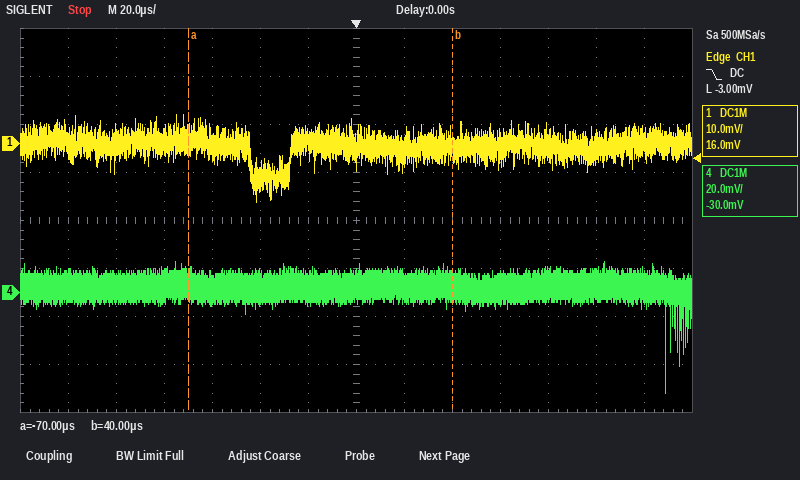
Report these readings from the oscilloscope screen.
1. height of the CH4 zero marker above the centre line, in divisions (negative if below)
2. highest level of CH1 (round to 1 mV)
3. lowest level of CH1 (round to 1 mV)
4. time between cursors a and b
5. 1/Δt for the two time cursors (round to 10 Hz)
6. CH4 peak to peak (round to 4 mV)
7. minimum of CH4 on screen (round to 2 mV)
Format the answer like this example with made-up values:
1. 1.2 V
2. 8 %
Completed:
1. -1.5 div
2. 6 mV
3. -12 mV
4. 110 µs
5. 9.09 kHz
6. 56 mV
7. -42 mV
